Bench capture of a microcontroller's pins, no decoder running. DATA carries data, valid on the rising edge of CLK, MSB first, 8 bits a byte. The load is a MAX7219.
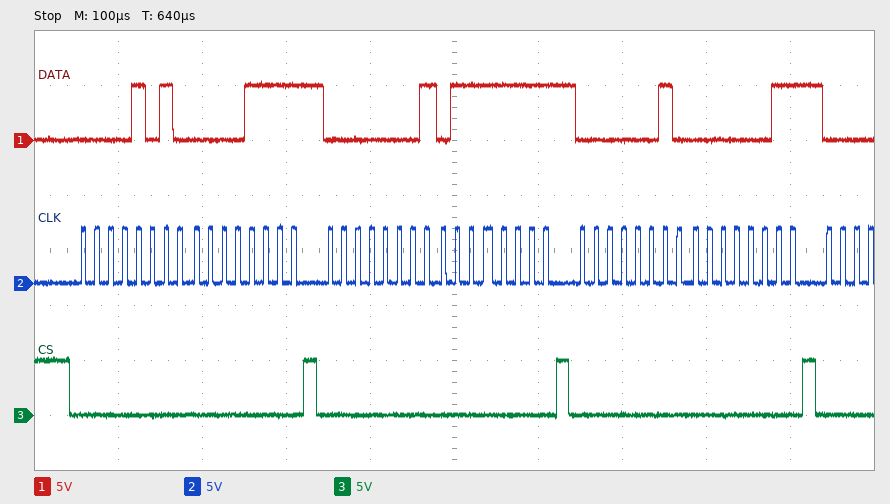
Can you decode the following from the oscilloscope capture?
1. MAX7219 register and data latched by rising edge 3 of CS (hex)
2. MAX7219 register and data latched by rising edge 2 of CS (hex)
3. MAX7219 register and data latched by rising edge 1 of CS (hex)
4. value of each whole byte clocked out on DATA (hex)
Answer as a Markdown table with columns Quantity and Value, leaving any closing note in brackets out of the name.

| Quantity | Value |
|---|---|
| MAX7219 register and data latched by rising edge 3 of CS | register 0x2, data 0x03 |
| MAX7219 register and data latched by rising edge 2 of CS | register 0x1, data 0x7F |
| MAX7219 register and data latched by rising edge 1 of CS | register 0xA, data 0x0F |
| value of each whole byte clocked out on DATA | 0A 0F 01 7F 02 03 |
